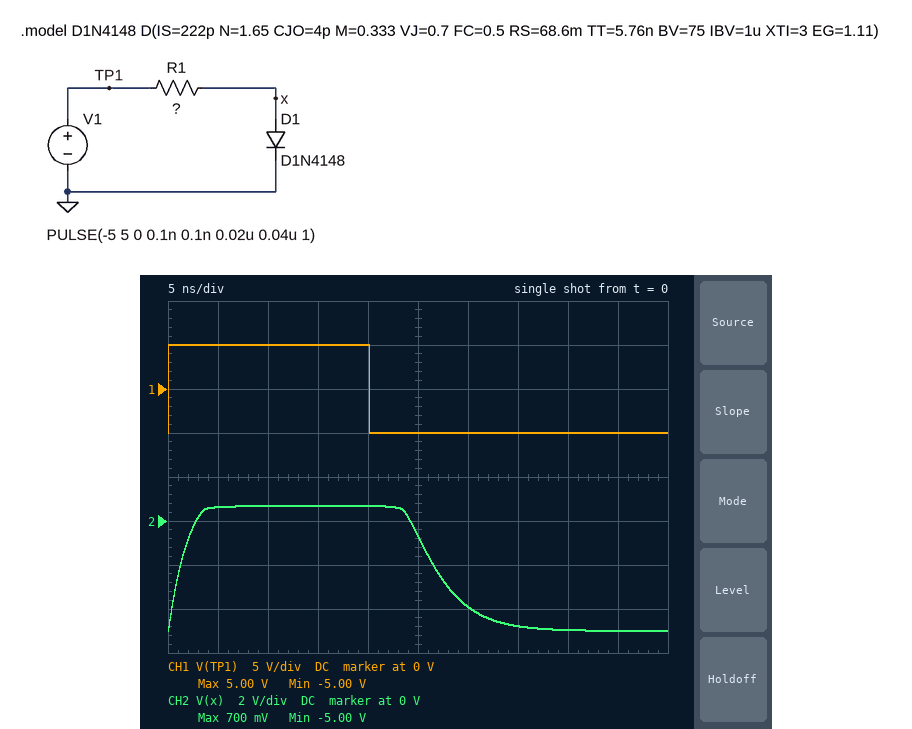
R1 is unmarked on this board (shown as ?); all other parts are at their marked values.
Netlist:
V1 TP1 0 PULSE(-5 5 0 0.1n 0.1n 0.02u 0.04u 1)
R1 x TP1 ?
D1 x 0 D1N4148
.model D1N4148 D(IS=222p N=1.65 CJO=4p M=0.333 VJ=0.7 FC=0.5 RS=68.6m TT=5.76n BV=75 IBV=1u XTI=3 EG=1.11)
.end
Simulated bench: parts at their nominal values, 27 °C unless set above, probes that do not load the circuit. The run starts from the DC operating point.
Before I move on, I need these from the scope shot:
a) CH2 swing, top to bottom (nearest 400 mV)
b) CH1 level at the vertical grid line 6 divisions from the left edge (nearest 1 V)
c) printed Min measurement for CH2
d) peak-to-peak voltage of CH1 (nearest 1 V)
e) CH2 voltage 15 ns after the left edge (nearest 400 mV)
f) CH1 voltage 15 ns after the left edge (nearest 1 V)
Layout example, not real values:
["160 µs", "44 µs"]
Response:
["5.6 V", "-5 V", "-5.00 V", "10 V", "800 mV", "5 V"]
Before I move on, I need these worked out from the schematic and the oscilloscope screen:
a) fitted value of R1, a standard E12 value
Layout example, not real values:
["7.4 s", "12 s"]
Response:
["1.5 kΩ"]
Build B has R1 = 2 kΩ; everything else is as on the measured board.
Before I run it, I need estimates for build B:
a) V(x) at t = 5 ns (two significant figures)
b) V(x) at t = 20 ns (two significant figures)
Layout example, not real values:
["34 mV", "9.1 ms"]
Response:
["540 mV", "680 mV"]
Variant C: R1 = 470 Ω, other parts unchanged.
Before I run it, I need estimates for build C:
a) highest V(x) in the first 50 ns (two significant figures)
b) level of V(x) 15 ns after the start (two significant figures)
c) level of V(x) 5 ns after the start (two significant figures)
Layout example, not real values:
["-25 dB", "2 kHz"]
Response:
["750 mV", "740 mV", "720 mV"]
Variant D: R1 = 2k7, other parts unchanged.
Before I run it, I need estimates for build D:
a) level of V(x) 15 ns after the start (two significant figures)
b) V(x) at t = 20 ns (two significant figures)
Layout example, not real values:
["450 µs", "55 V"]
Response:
["660 mV", "670 mV"]
